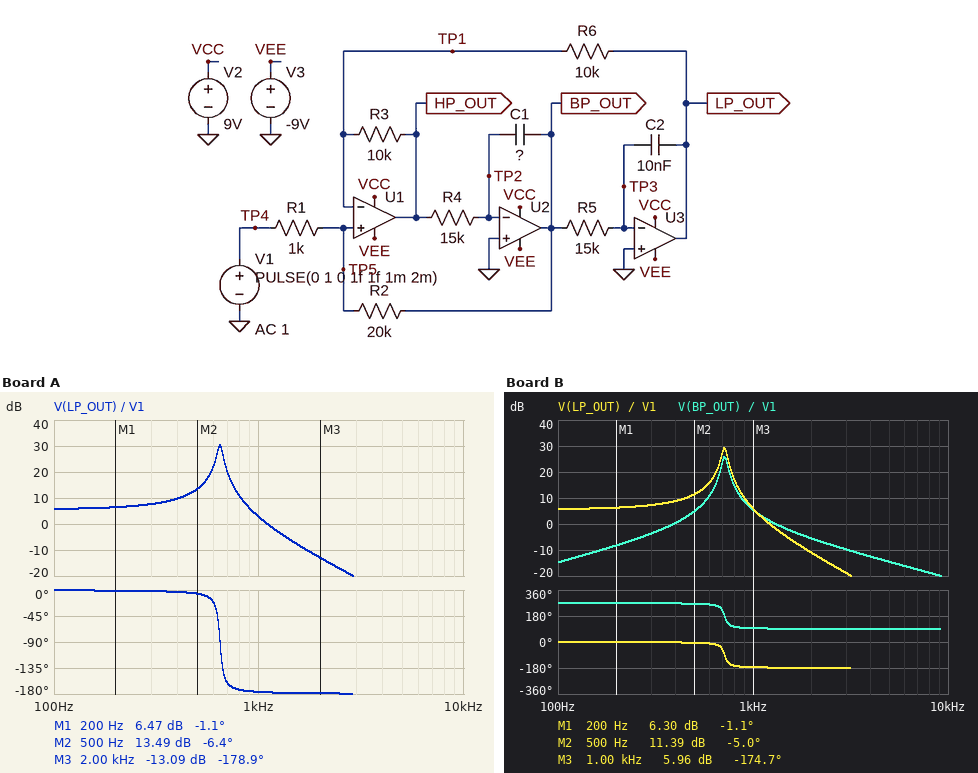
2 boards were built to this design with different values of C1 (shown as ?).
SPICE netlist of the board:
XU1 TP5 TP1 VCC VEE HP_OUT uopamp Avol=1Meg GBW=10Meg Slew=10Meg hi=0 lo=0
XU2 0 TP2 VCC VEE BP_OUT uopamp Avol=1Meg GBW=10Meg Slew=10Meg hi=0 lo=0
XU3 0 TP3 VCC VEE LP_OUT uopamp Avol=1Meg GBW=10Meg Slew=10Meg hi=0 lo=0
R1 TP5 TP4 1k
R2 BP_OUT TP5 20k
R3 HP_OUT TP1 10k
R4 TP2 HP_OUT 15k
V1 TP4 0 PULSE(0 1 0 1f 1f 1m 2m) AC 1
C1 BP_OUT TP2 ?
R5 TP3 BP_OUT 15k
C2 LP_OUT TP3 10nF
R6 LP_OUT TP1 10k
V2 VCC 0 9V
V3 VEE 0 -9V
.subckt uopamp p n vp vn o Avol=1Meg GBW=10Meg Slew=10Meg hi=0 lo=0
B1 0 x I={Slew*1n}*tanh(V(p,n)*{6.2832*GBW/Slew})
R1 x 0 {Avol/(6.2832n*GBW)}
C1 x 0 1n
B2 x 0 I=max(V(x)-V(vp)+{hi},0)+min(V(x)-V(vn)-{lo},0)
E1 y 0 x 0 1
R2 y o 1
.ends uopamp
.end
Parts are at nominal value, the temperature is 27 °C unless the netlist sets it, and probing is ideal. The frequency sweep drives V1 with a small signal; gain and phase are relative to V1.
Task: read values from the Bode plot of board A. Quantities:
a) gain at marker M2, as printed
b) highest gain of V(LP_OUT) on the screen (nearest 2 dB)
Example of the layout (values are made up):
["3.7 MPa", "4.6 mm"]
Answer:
["13.49 dB", "30 dB"]
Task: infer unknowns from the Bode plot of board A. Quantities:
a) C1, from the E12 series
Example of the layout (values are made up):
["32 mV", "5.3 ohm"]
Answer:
["27 nF"]
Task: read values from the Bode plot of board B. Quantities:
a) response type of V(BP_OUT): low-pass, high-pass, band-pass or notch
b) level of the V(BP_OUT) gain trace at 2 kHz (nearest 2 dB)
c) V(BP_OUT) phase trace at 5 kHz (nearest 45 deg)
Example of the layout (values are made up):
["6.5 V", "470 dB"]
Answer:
["band-pass", "-6 dB", "90 deg"]
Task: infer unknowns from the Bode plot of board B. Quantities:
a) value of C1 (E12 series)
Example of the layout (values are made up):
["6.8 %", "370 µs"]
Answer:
["22 nF"]
